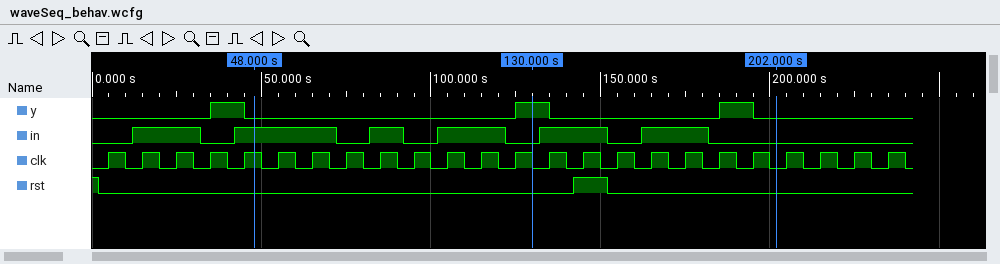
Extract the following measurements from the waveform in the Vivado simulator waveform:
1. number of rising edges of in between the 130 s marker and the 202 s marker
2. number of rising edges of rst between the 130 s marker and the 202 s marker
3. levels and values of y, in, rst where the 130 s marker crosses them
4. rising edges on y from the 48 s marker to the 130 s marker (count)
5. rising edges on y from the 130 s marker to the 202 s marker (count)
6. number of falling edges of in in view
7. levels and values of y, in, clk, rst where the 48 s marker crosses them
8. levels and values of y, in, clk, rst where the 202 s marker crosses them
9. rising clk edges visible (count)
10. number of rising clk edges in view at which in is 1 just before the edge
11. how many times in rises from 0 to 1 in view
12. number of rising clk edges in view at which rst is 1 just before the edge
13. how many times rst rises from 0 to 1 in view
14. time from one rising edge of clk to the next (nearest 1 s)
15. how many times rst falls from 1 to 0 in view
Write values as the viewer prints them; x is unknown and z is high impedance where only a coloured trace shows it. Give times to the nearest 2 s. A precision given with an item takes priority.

2
1
y=1, in=0, rst=0
1
1
6
y=0, in=1, clk=1, rst=0
y=0, in=0, clk=0, rst=0
24
12
6
1
1
10 s
2
